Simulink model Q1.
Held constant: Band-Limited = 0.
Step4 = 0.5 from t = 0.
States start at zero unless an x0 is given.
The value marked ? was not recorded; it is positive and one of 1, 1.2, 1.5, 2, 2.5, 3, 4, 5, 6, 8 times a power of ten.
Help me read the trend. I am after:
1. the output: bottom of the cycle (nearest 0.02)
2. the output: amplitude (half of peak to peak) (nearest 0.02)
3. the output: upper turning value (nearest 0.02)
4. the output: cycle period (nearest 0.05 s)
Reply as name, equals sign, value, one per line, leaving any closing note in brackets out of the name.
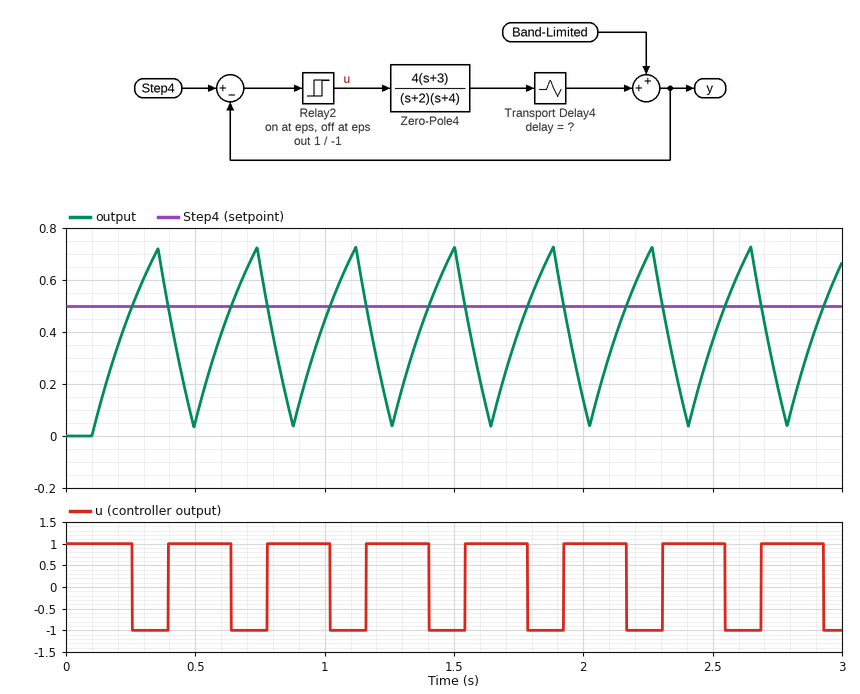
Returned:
the output: bottom of the cycle = 0.04
the output: amplitude (half of peak to peak) = 0.34
the output: upper turning value = 0.72
the output: cycle period = 0.40 s
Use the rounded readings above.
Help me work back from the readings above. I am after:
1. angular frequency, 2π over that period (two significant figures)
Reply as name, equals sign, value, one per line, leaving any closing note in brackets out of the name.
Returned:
angular frequency, 2π over that period = 16 rad/s
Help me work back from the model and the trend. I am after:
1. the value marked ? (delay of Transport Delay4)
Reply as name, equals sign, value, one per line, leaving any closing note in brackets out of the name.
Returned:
the value marked ? = 0.1
